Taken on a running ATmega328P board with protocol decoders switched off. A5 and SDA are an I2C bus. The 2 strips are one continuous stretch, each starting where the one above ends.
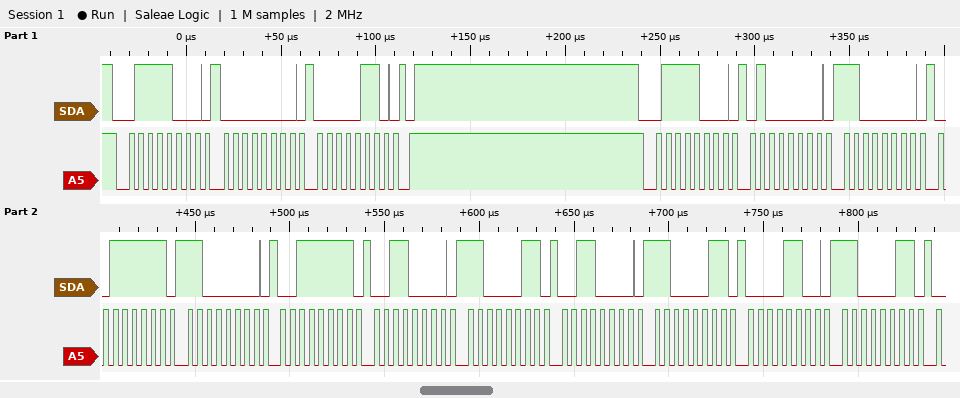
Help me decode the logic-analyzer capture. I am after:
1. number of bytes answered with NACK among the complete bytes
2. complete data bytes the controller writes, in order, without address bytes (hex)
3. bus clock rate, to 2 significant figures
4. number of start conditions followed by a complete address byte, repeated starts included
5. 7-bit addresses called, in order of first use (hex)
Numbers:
0
00 06 40 C0 3F C0 3F 30 C3 30 C3 0C C3
200 kHz
2
0x3C
